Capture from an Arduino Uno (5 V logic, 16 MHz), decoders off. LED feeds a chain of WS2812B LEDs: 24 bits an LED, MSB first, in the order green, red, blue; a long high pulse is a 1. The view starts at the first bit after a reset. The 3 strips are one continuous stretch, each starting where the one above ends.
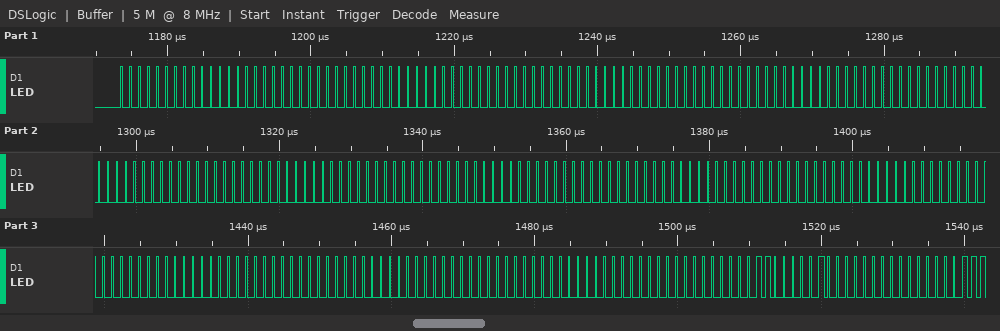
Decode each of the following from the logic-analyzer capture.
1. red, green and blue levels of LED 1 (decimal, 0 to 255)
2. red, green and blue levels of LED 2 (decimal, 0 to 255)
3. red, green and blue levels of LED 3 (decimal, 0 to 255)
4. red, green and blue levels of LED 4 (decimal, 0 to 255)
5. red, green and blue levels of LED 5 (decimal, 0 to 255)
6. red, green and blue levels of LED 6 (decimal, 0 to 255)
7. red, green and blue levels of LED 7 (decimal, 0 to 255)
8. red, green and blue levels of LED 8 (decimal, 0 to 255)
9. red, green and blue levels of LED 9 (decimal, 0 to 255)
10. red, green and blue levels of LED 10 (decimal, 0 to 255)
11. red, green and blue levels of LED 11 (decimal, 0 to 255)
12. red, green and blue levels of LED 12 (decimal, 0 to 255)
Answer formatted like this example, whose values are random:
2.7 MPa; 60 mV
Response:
0, 0, 0; 0, 0, 0; 0, 0, 0; 0, 0, 0; 0, 0, 0; 0, 0, 0; 0, 0, 0; 0, 0, 0; 0, 0, 0; 0, 0, 0; 0, 0, 0; 4, 3, 0
